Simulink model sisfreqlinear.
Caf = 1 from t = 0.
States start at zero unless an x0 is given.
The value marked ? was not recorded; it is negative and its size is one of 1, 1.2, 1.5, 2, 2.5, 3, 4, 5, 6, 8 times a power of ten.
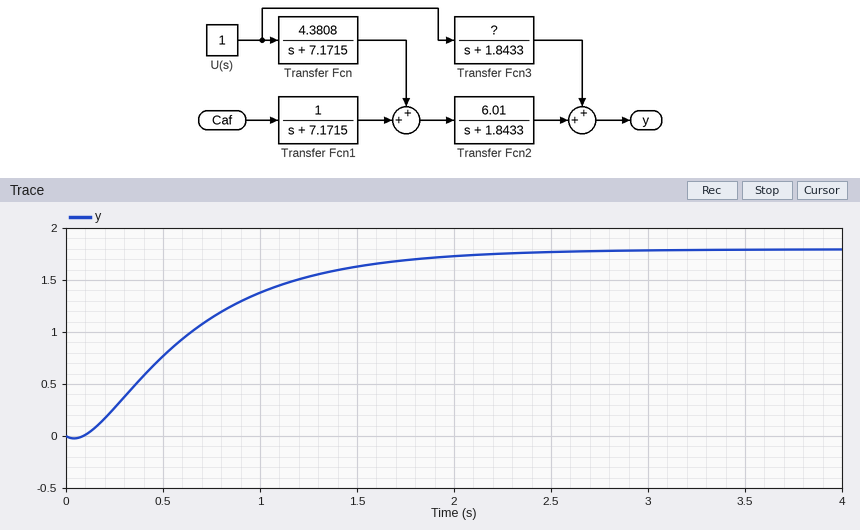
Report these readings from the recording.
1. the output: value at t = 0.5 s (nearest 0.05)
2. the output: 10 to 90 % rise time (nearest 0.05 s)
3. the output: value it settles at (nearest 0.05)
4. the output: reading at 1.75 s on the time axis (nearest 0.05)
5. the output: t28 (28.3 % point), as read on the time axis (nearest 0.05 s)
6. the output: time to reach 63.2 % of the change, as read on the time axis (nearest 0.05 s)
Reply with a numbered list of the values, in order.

1. 0.75
2. 1.25 s
3. 1.80
4. 1.70
5. 0.35 s
6. 0.75 s
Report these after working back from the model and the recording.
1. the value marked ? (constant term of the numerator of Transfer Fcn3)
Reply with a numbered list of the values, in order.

1. -1.2
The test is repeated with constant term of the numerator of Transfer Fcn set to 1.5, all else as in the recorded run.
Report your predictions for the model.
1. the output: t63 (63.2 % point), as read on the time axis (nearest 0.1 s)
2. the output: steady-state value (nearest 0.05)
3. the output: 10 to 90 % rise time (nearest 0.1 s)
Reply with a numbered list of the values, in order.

1. 0.9 s
2. 0.50
3. 1.2 s
